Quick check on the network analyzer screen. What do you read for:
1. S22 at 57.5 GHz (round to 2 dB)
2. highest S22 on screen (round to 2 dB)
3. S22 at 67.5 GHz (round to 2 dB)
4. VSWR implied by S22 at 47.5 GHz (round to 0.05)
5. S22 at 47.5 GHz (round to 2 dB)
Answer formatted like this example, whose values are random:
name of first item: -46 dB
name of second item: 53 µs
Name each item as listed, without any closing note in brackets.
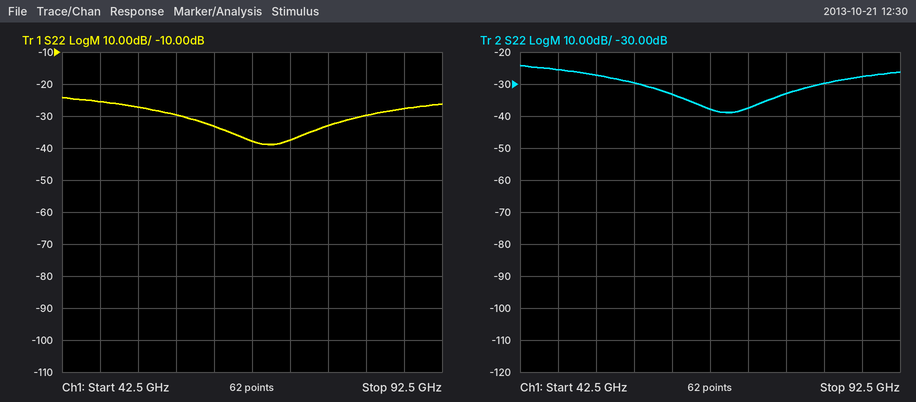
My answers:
S22 at 57.5 GHz: -30 dB
highest S22 on screen: -24 dB
S22 at 67.5 GHz: -38 dB
VSWR implied by S22 at 47.5 GHz: 1.10
S22 at 47.5 GHz: -26 dB
